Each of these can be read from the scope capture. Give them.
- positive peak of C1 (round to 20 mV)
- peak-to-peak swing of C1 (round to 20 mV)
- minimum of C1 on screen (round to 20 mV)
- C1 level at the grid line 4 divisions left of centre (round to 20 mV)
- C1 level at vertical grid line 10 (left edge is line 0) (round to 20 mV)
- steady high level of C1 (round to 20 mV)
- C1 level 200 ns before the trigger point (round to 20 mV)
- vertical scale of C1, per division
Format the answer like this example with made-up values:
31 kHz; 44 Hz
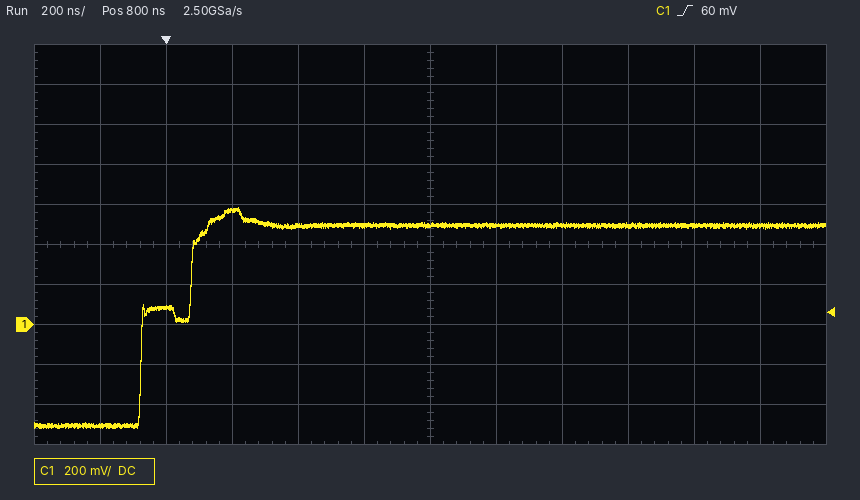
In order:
580 mV; 1.10 V; -520 mV; 80 mV; 500 mV; 500 mV; -500 mV; 200 mV
